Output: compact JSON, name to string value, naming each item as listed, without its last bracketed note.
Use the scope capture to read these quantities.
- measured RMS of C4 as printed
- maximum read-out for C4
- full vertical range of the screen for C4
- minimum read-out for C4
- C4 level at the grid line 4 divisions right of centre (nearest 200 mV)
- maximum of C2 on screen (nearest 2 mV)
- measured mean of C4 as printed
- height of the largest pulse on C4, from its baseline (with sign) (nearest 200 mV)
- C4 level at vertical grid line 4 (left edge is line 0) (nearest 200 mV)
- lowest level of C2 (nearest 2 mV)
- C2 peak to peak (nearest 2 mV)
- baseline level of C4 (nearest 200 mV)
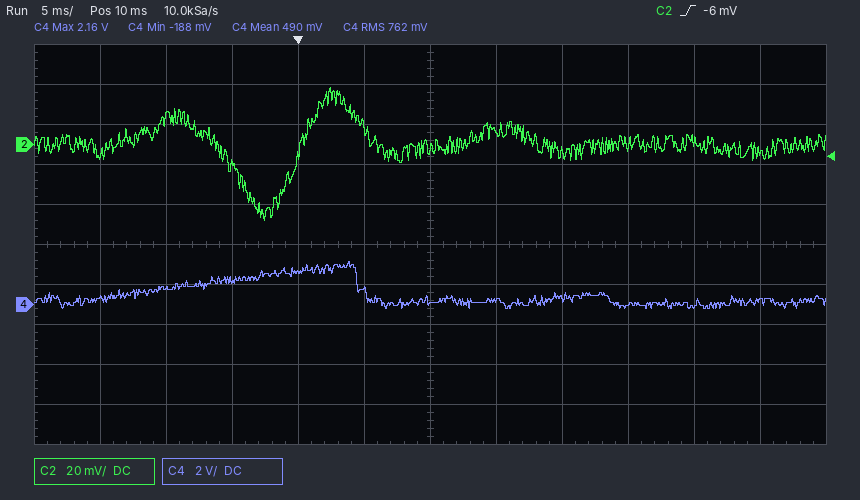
{"measured RMS of C4 as printed": "762 mV", "maximum read-out for C4": "2.16 V", "full vertical range of the screen for C4": "20 V", "minimum read-out for C4": "-188 mV", "C4 level at the grid line 4 divisions right of centre": "0.0 V", "maximum of C2 on screen": "28 mV", "measured mean of C4 as printed": "490 mV", "height of the largest pulse on C4, from its baseline (with sign)": "+2.0 V", "C4 level at vertical grid line 4 (left edge is line 0)": "1.6 V", "lowest level of C2": "-38 mV", "C2 peak to peak": "66 mV", "baseline level of C4": "200 mV"}
